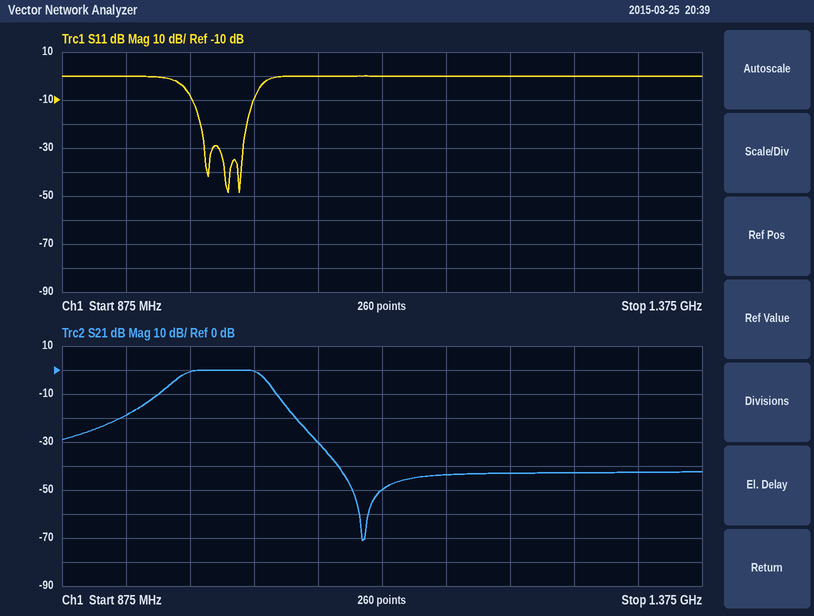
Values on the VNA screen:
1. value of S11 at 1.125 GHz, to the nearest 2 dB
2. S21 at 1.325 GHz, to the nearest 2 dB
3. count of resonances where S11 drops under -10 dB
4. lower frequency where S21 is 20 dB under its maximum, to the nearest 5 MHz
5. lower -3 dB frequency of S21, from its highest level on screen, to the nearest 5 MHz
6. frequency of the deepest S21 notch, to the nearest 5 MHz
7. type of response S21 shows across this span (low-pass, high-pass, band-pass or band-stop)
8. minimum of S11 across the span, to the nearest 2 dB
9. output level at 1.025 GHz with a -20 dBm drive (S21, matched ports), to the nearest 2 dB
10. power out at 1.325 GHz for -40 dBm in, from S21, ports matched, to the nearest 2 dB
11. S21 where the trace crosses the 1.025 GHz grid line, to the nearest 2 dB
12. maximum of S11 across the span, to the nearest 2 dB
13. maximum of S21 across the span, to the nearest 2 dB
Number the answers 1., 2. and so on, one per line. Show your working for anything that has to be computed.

1. 0 dB
2. -42 dB
3. 3
4. 920 MHz
5. 965 MHz
6. 1.110 GHz
7. band-pass
8. -48 dB
9. -20 dBm + (0 dB) = -20 dBm
10. -40 dBm + (-42 dB) = -82 dBm
11. 0 dB
12. 0 dB
13. 0 dB
